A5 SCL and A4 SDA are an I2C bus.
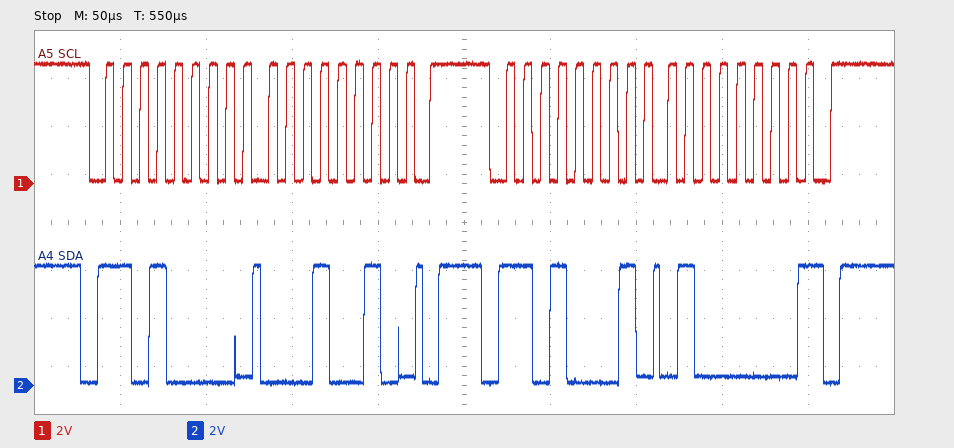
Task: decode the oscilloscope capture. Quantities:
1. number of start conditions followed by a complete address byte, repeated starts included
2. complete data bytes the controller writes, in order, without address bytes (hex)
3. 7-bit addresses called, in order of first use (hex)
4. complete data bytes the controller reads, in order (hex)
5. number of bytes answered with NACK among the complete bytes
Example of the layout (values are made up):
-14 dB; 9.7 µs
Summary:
2; 12; 0x68; 40; 1
